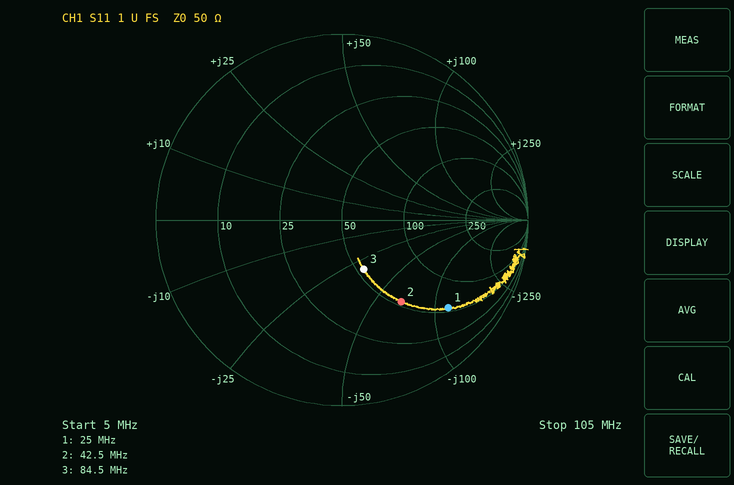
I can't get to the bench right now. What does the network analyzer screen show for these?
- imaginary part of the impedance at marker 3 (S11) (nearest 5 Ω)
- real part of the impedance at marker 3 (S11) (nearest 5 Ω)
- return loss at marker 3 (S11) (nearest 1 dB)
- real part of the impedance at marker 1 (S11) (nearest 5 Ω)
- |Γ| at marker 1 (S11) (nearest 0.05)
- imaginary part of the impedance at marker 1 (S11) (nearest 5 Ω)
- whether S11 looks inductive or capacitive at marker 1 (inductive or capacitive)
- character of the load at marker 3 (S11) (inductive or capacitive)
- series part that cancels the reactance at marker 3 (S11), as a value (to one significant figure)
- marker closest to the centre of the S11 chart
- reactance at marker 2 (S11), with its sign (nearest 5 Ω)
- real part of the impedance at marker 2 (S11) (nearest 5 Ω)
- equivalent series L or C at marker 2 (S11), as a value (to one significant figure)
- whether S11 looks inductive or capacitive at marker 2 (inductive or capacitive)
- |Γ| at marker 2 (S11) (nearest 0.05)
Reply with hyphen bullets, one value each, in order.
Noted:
- -30 Ω
- 55 Ω
- 11 dB
- 55 Ω
- 0.75
- -115 Ω
- capacitive
- capacitive
- 60 nH
- marker 3
- -65 Ω
- 55 Ω
- 60 pF
- capacitive
- 0.55
